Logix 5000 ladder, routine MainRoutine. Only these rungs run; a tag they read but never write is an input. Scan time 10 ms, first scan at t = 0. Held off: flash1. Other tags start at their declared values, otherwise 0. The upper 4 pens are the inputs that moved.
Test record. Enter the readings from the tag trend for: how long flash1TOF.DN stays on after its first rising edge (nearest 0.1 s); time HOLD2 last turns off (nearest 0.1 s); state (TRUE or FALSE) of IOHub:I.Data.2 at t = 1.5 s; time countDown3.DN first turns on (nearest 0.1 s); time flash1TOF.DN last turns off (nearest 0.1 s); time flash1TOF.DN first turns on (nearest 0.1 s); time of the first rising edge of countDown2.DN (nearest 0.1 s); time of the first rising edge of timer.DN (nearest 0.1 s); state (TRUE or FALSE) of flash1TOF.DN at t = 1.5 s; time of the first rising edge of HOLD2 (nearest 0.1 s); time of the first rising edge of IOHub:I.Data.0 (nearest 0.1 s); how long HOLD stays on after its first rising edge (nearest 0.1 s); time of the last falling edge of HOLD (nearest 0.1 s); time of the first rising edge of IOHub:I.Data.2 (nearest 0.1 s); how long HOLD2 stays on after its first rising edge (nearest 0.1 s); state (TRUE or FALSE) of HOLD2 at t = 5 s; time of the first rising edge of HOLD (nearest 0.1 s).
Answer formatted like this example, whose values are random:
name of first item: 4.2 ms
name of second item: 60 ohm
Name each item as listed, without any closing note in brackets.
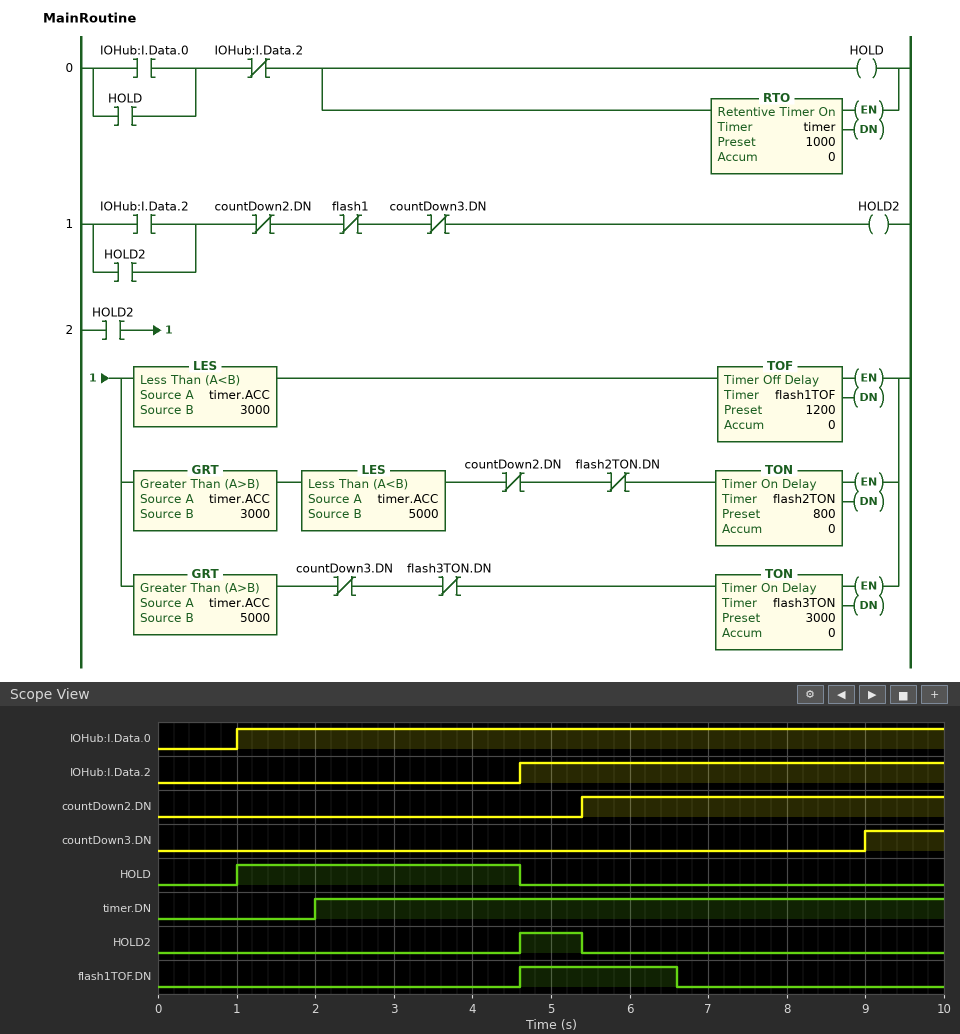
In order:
how long flash1TOF.DN stays on after its first rising edge: 2.0 s
time HOLD2 last turns off: 5.4 s
state (TRUE or FALSE) of IOHub:I.Data.2 at t = 1.5 s: FALSE
time countDown3.DN first turns on: 9.0 s
time flash1TOF.DN last turns off: 6.6 s
time flash1TOF.DN first turns on: 4.6 s
time of the first rising edge of countDown2.DN: 5.4 s
time of the first rising edge of timer.DN: 2.0 s
state (TRUE or FALSE) of flash1TOF.DN at t = 1.5 s: FALSE
time of the first rising edge of HOLD2: 4.6 s
time of the first rising edge of IOHub:I.Data.0: 1.0 s
how long HOLD stays on after its first rising edge: 3.6 s
time of the last falling edge of HOLD: 4.6 s
time of the first rising edge of IOHub:I.Data.2: 4.6 s
how long HOLD2 stays on after its first rising edge: 0.8 s
state (TRUE or FALSE) of HOLD2 at t = 5 s: TRUE
time of the first rising edge of HOLD: 1.0 s
